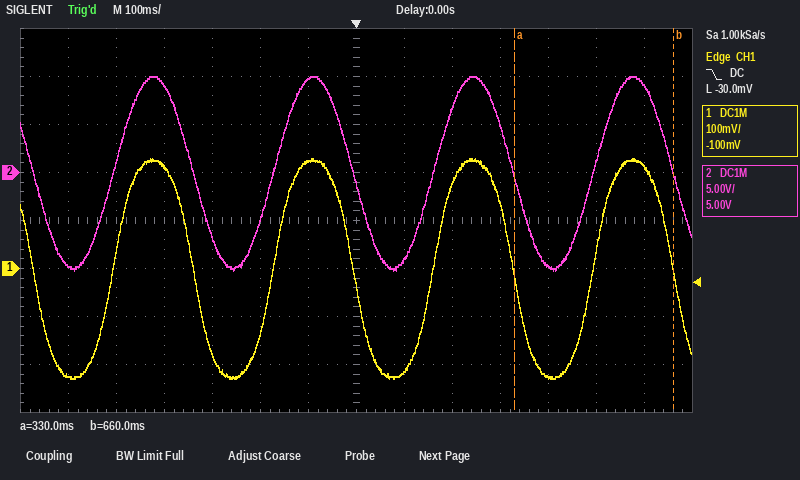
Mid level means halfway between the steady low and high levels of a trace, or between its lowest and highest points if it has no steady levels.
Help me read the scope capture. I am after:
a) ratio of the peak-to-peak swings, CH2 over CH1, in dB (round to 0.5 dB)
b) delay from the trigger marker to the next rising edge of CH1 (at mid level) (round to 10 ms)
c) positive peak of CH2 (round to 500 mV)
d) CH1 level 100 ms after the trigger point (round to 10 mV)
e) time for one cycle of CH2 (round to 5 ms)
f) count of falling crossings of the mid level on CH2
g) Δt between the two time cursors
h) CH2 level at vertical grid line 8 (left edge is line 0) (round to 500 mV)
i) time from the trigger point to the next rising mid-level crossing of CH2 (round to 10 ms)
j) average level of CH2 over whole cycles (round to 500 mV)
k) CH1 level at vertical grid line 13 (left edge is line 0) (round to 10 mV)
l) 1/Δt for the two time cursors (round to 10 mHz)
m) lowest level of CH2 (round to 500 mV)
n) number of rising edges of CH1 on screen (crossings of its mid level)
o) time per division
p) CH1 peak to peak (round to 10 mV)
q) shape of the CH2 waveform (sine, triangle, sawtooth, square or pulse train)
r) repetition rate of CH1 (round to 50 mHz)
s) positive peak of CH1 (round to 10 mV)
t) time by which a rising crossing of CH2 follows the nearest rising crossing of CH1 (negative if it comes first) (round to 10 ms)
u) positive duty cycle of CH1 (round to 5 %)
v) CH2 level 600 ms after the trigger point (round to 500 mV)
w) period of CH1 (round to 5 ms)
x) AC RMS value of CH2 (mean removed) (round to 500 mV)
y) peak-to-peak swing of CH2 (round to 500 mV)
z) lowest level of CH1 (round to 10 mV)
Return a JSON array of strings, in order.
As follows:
["33.0 dB", "160 ms", "10.0 V", "-210 mV", "335 ms", "5", "330 ms", "-9.0 V", "160 ms", "0.0 V", "210 mV", "3.03 Hz", "-10.0 V", "4", "100 ms", "460 mV", "sine", "3.00 Hz", "230 mV", "0 ms", "50 %", "9.0 V", "335 ms", "7.0 V", "20.0 V", "-230 mV"]
